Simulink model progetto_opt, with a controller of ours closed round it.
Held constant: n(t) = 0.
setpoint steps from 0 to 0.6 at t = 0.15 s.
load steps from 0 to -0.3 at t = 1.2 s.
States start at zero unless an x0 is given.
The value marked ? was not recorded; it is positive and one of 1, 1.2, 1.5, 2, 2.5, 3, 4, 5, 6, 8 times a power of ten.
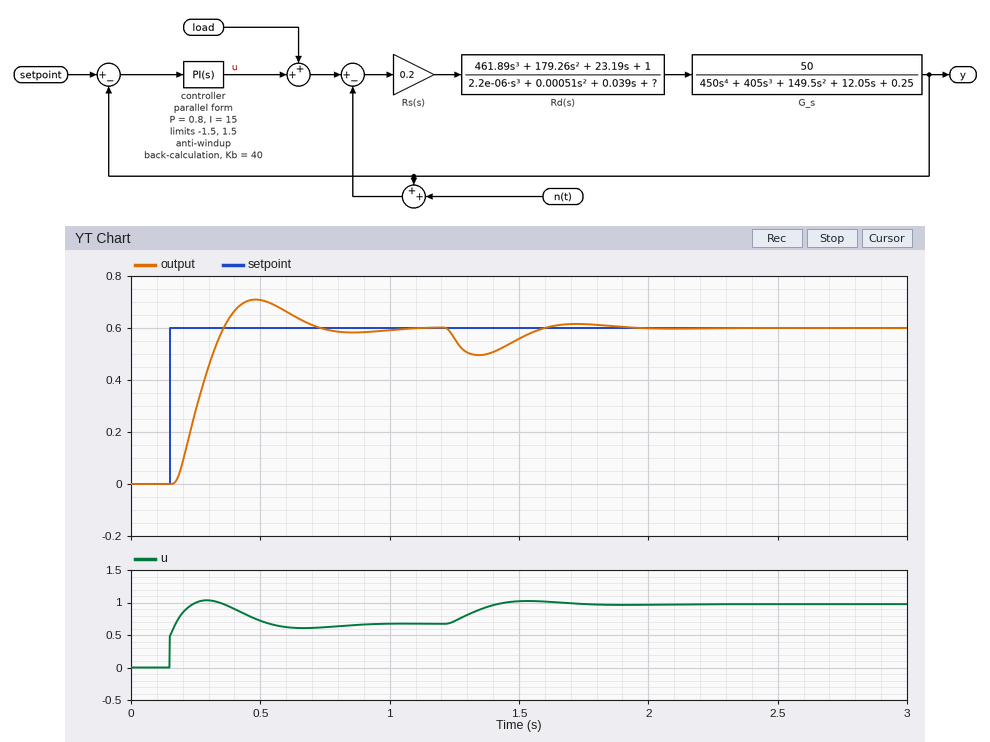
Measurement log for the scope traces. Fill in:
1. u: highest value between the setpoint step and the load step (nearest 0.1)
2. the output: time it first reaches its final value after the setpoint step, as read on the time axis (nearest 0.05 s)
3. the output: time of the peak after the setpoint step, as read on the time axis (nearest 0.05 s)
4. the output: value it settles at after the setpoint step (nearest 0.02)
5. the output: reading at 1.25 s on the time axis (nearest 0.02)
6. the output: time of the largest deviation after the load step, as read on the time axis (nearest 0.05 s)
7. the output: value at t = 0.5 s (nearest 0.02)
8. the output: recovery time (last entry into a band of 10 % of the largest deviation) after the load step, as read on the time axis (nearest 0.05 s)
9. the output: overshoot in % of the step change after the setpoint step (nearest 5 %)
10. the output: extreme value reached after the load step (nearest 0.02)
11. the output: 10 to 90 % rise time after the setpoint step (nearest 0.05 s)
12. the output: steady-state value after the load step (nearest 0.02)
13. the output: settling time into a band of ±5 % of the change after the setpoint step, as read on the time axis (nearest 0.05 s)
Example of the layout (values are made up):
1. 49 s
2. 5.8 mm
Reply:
1. 1.0
2. 0.35 s
3. 0.50 s
4. 0.60
5. 0.56
6. 1.35 s
7. 0.70
8. 1.80 s
9. 20 %
10. 0.50
11. 0.15 s
12. 0.60
13. 0.65 s
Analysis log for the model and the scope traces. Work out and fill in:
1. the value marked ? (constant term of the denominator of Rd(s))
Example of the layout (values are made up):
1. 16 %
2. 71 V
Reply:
1. 2
